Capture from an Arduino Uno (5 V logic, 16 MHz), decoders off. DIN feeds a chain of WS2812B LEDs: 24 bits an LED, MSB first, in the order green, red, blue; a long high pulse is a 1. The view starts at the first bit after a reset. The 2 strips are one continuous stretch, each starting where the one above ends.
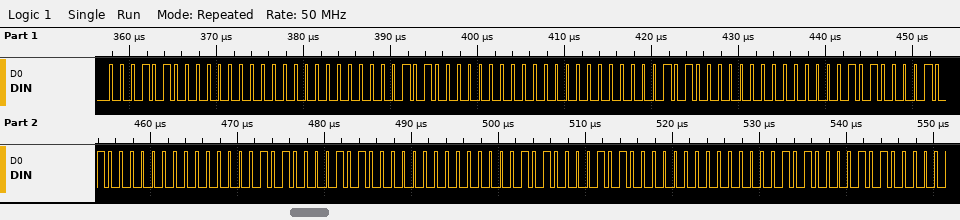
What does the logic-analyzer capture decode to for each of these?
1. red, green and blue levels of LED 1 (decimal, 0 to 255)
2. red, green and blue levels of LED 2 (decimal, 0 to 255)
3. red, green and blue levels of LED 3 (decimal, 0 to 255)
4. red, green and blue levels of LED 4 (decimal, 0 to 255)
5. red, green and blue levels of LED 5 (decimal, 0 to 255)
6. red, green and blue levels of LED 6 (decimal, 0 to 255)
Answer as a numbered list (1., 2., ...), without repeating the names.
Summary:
1. 0, 20, 0
2. 0, 20, 0
3. 0, 20, 10
4. 0, 20, 10
5. 0, 20, 10
6. 0, 20, 10
